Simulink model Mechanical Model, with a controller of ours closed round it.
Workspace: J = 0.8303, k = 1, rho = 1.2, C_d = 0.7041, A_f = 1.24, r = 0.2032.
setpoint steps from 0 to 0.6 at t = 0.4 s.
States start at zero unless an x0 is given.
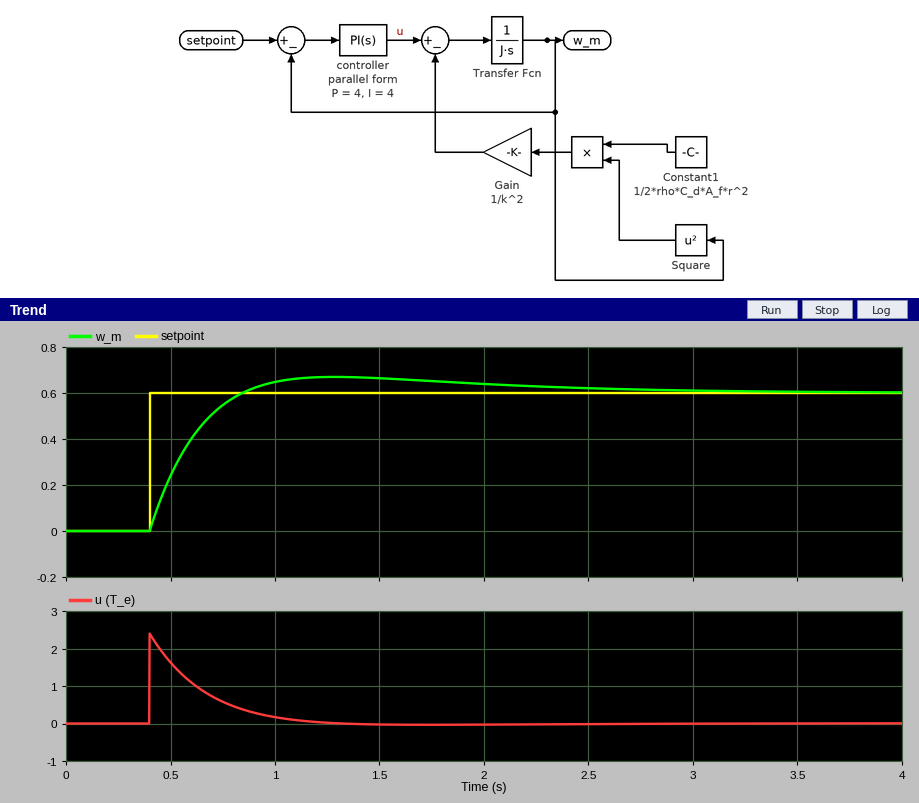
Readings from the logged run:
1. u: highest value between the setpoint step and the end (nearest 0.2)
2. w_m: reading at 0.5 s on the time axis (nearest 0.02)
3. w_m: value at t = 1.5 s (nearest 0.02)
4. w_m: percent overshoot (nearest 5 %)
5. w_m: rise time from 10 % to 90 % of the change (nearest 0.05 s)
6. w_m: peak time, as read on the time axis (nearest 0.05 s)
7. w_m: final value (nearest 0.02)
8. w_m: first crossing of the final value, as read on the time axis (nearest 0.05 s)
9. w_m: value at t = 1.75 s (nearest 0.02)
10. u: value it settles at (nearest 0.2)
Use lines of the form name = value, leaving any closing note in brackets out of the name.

u: highest value between the setpoint step and the end = 2.4
w_m: reading at 0.5 s on the time axis = 0.24
w_m: value at t = 1.5 s = 0.66
w_m: percent overshoot = 10 %
w_m: rise time from 10 % to 90 % of the change = 0.30 s
w_m: peak time, as read on the time axis = 1.30 s
w_m: final value = 0.60
w_m: first crossing of the final value, as read on the time axis = 0.85 s
w_m: value at t = 1.75 s = 0.66
u: value it settles at = 0.0
